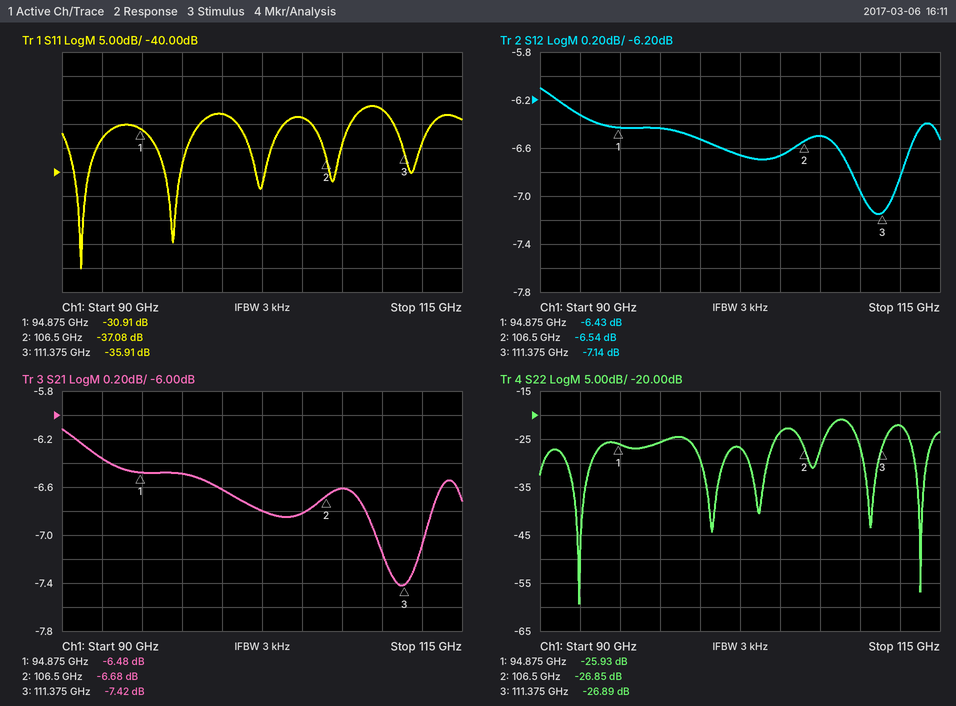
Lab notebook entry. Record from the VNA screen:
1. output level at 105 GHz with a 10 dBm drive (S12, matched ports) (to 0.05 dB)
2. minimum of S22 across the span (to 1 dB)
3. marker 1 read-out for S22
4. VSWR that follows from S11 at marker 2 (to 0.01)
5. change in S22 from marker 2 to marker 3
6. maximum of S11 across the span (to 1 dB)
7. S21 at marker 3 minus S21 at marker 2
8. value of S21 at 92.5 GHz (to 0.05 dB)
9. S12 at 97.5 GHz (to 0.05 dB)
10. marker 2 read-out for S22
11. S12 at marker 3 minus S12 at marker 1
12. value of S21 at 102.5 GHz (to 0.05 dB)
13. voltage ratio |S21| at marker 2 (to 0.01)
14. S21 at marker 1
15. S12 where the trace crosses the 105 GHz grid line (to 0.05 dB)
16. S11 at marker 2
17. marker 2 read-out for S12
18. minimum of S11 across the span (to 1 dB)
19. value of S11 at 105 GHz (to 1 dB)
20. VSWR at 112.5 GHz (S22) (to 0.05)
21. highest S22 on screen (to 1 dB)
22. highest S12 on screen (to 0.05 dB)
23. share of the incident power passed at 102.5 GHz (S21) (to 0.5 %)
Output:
3.35 dBm
-59 dB
-25.93 dB
1.03
-0.04 dB
-26 dB
-0.74 dB
-6.35 dB
-6.45 dB
-26.85 dB
-0.71 dB
-6.80 dB
0.46
-6.48 dB
-6.65 dB
-37.08 dB
-6.54 dB
-60 dB
-29 dB
1.15
-21 dB
-6.10 dB
21.0 %
